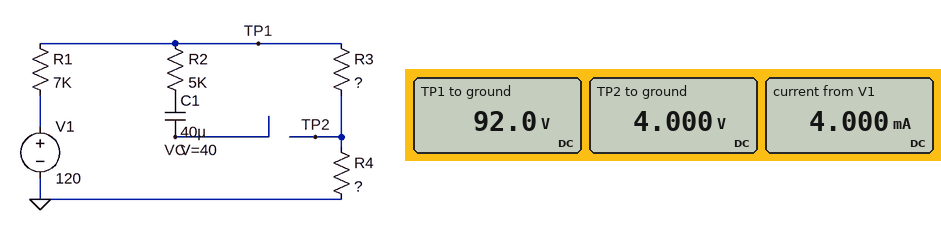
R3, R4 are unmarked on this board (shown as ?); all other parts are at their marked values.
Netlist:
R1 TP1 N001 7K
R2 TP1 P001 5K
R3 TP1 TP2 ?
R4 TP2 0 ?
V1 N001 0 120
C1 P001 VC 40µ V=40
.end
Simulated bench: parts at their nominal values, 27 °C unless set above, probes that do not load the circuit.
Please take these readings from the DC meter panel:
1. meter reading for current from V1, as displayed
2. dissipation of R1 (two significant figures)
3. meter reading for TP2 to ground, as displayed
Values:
4.000 mA
110 mW
4.000 V
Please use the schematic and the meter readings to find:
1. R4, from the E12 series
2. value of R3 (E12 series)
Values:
1 kΩ
22 kΩ
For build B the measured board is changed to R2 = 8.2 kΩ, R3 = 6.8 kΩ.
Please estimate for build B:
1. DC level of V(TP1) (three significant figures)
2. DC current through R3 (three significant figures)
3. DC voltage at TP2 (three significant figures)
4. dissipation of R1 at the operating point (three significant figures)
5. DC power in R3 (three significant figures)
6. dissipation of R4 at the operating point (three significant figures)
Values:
63.2 V
8.11 mA
8.11 V
460 mW
447 mW
65.7 mW
